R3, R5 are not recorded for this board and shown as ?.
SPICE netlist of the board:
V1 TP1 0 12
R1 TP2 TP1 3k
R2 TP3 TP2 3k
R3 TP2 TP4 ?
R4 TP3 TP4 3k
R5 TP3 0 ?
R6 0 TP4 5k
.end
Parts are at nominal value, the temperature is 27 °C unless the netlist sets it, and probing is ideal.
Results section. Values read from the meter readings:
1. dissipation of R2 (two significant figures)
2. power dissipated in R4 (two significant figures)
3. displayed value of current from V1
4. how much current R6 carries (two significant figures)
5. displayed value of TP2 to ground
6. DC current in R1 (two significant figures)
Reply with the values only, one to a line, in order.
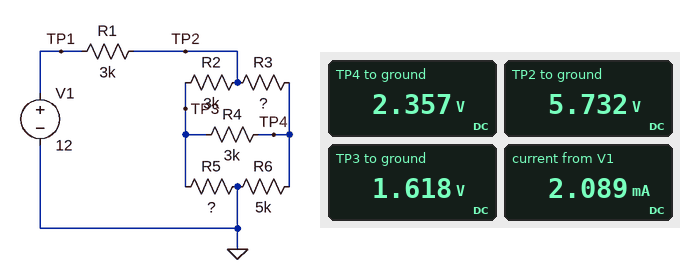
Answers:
5.6 mW
180 µW
2.089 mA
470 µA
5.732 V
2.1 mA
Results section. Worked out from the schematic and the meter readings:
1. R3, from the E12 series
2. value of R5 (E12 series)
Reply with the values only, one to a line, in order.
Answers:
4.7 kΩ
1 kΩ
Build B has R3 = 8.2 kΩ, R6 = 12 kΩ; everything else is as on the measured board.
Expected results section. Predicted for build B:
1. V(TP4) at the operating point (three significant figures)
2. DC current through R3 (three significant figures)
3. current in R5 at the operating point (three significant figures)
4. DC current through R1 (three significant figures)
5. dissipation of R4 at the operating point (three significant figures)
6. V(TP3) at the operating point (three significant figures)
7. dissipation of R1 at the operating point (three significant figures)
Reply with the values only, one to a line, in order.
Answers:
2.47 V
453 µA
1.73 mA
1.94 mA
183 µW
1.73 V
11.3 mW
